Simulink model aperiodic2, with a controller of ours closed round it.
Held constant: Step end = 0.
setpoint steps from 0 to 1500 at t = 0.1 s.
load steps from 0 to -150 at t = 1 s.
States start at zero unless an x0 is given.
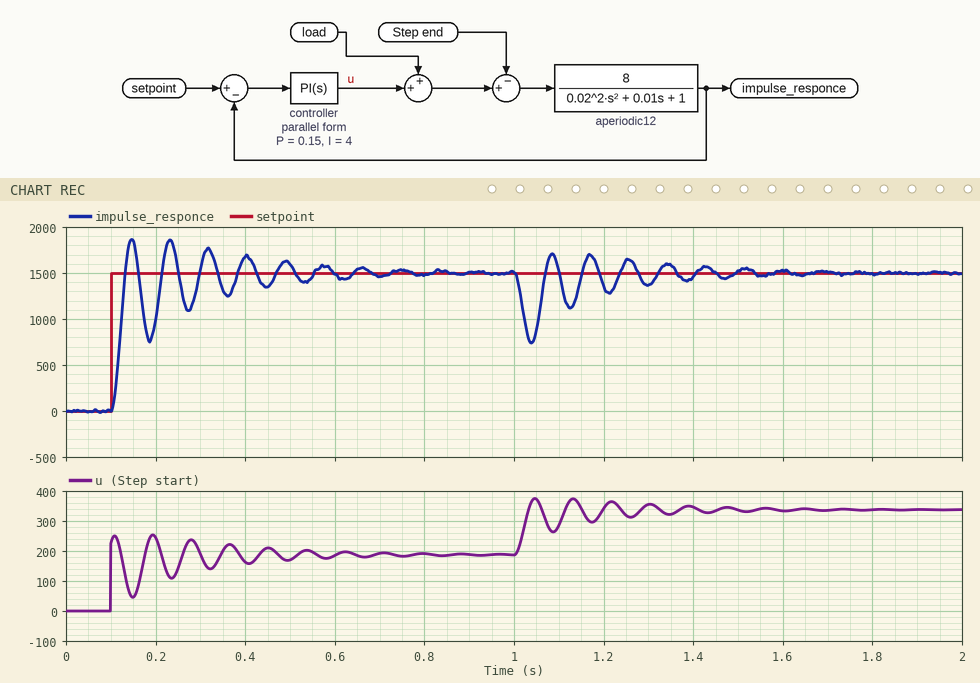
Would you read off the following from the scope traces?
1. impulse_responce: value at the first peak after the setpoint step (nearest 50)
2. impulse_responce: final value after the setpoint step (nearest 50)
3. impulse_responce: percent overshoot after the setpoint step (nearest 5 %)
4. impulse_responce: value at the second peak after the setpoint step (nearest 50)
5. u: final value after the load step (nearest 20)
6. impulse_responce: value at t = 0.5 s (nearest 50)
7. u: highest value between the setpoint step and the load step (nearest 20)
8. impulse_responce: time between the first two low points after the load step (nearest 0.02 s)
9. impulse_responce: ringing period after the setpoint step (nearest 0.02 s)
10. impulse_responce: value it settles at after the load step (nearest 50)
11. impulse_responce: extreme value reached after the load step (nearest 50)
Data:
1850
1500
25 %
1850
340
1600
260
0.08 s
0.08 s
1500
750
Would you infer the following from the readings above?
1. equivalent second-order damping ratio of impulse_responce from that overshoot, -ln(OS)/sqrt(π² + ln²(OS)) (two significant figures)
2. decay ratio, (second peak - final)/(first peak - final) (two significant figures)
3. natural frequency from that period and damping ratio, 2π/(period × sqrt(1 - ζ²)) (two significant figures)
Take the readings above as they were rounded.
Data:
0.40
1.0
86 rad/s
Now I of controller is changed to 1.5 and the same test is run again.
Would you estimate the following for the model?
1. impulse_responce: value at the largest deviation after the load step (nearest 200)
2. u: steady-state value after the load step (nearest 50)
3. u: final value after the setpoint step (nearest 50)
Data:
600
350
200
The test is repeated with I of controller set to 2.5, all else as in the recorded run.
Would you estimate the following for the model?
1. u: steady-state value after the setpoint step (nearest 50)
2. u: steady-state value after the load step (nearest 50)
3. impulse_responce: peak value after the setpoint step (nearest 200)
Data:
200
350
1600
